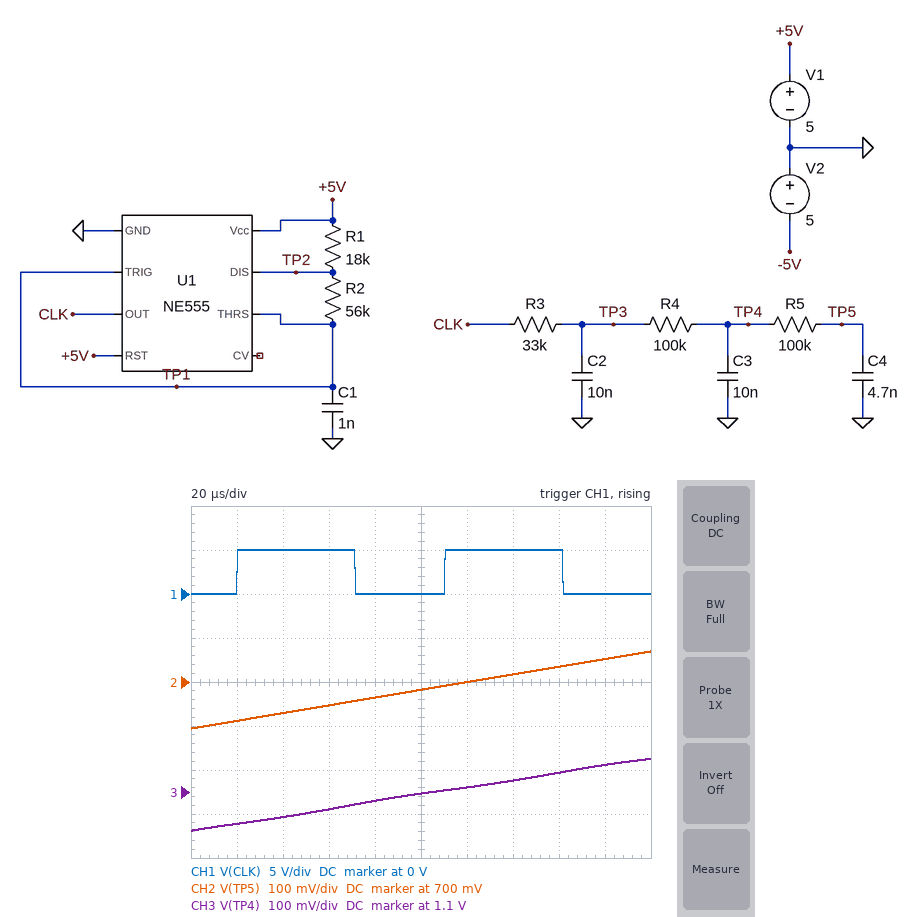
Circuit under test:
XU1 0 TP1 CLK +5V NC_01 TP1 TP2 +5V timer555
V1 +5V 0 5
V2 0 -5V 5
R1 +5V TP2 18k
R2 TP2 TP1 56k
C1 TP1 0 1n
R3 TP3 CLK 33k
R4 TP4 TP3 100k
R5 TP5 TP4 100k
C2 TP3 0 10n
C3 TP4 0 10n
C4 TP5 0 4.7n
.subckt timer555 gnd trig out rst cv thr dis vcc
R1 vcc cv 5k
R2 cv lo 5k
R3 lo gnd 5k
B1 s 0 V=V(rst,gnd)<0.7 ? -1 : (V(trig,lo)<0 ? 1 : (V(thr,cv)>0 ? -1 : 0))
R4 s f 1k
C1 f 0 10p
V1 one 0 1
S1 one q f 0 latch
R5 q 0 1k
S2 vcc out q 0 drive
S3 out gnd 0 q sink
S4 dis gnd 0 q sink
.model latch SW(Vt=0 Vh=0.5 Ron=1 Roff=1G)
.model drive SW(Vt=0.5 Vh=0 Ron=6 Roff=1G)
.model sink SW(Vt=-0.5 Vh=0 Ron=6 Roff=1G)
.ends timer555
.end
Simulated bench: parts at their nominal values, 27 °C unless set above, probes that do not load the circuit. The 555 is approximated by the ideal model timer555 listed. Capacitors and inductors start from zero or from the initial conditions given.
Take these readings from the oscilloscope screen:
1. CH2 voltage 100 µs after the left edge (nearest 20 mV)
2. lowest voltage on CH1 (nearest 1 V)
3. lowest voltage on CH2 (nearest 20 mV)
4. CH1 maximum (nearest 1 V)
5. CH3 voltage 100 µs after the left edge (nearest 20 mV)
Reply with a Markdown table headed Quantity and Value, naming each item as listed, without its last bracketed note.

| Quantity | Value |
|---|---|
| CH2 voltage 100 µs after the left edge | 680 mV |
| lowest voltage on CH1 | 0 V |
| lowest voltage on CH2 | 600 mV |
| CH1 maximum | 5 V |
| CH3 voltage 100 µs after the left edge | 1.10 V |
